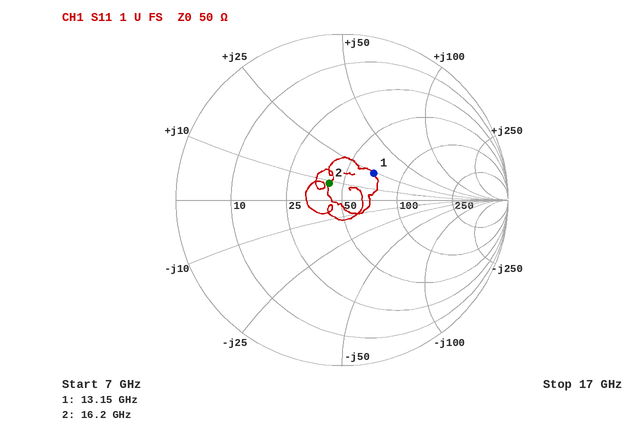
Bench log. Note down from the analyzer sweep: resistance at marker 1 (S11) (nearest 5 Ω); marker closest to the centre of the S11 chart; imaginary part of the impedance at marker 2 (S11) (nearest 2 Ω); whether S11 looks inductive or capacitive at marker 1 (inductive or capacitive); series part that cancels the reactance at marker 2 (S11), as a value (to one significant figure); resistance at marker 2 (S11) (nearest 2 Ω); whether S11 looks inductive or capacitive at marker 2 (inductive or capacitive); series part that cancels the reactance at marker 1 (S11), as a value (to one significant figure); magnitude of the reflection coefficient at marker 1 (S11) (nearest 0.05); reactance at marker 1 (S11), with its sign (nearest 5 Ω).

70 Ω
marker 2
+8 Ω
inductive
1 pF
42 Ω
inductive
500 fF
0.25
+25 Ω
